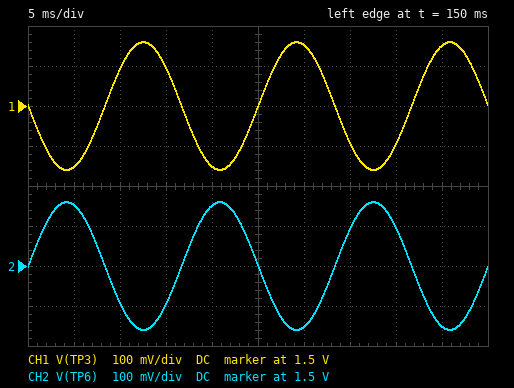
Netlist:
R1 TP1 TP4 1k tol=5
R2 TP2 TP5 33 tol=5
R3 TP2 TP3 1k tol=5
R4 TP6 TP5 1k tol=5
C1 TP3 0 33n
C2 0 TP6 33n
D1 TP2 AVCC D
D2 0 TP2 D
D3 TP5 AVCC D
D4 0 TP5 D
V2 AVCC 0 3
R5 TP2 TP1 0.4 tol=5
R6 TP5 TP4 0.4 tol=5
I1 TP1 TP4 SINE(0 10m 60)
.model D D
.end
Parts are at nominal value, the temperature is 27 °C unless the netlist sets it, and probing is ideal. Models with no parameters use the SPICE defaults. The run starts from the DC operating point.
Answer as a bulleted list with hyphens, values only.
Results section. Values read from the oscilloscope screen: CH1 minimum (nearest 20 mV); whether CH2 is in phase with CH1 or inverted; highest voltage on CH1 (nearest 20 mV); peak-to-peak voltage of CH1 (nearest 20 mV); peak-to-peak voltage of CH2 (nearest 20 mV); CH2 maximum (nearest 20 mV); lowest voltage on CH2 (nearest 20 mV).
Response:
- 1.34 V
- inverted
- 1.66 V
- 320 mV
- 320 mV
- 1.66 V
- 1.34 V
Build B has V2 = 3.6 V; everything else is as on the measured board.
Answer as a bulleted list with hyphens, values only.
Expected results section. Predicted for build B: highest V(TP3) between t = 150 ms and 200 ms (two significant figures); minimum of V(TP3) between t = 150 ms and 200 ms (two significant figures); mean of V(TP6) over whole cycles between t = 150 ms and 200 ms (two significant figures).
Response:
- 2.0 V
- 1.6 V
- 1.8 V
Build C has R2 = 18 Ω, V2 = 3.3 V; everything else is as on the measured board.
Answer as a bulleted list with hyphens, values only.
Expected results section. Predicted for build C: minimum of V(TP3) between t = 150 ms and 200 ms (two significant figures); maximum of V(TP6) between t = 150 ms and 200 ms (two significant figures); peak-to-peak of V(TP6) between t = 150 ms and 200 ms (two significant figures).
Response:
- 1.6 V
- 1.7 V
- 180 mV
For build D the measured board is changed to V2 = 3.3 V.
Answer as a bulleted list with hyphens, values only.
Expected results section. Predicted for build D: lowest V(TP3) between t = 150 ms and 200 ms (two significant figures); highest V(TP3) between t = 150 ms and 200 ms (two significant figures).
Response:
- 1.5 V
- 1.8 V
